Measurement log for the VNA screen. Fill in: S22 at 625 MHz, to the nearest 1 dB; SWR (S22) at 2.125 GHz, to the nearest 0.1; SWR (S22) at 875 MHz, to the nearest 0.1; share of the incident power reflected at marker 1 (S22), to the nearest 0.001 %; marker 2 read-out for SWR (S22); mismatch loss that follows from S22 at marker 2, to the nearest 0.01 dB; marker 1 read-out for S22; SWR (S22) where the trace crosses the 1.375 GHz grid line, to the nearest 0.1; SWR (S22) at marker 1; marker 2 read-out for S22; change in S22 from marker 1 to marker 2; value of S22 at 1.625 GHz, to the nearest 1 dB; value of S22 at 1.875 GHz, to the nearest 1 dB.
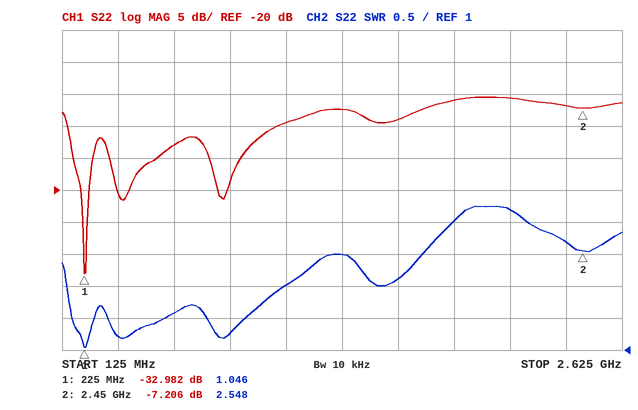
-13 dB
3.2
1.3
0.050 %
2.548
0.92 dB
-32.982 dB
2.5
1.046
-7.206 dB
25.776 dB
-9 dB
-6 dB
